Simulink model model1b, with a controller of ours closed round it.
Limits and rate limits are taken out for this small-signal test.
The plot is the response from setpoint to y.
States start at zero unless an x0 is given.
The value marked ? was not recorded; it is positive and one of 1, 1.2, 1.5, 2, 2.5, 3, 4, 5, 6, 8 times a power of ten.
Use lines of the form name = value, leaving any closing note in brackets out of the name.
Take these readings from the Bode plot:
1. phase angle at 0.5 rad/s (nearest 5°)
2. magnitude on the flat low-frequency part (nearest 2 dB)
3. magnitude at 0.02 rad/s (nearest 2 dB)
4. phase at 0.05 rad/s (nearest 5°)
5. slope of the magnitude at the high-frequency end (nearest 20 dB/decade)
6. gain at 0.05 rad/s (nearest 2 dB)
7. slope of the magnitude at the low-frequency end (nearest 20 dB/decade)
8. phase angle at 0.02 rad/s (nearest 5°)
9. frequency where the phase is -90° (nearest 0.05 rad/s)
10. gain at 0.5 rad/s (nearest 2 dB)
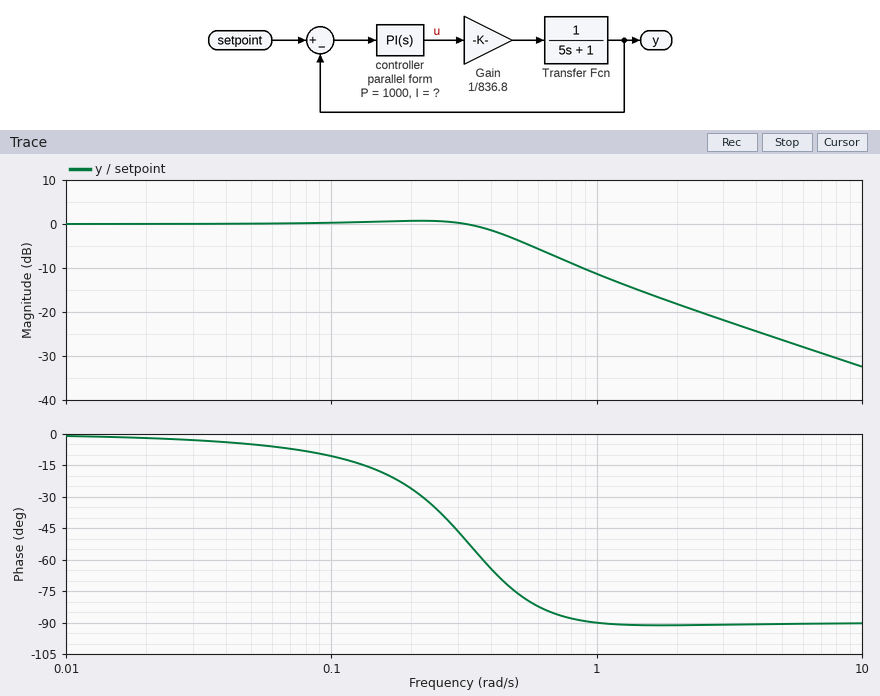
phase angle at 0.5 rad/s = -75°
magnitude on the flat low-frequency part = 0 dB
magnitude at 0.02 rad/s = 0 dB
phase at 0.05 rad/s = -5°
slope of the magnitude at the high-frequency end = -20 dB/decade
gain at 0.05 rad/s = 0 dB
slope of the magnitude at the low-frequency end = 0 dB/decade
phase angle at 0.02 rad/s = 0°
frequency where the phase is -90° = 1.00 rad/s
gain at 0.5 rad/s = -4 dB
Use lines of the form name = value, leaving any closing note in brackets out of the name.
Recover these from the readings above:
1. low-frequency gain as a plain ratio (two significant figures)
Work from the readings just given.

low-frequency gain as a plain ratio = 1.0
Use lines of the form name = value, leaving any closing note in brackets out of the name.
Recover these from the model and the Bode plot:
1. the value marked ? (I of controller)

the value marked ? = 500
